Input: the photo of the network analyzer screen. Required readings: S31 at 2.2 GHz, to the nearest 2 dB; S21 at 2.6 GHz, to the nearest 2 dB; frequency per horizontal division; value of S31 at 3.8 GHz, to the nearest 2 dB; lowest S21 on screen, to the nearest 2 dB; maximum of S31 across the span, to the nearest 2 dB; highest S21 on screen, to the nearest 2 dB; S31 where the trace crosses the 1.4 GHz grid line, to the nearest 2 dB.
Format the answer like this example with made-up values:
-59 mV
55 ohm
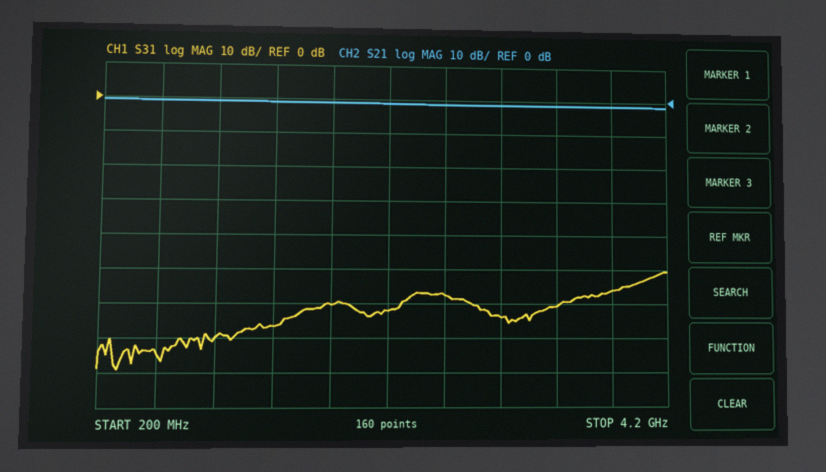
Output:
-62 dB
-2 dB
400 MHz
-56 dB
-2 dB
-50 dB
0 dB
-66 dB
